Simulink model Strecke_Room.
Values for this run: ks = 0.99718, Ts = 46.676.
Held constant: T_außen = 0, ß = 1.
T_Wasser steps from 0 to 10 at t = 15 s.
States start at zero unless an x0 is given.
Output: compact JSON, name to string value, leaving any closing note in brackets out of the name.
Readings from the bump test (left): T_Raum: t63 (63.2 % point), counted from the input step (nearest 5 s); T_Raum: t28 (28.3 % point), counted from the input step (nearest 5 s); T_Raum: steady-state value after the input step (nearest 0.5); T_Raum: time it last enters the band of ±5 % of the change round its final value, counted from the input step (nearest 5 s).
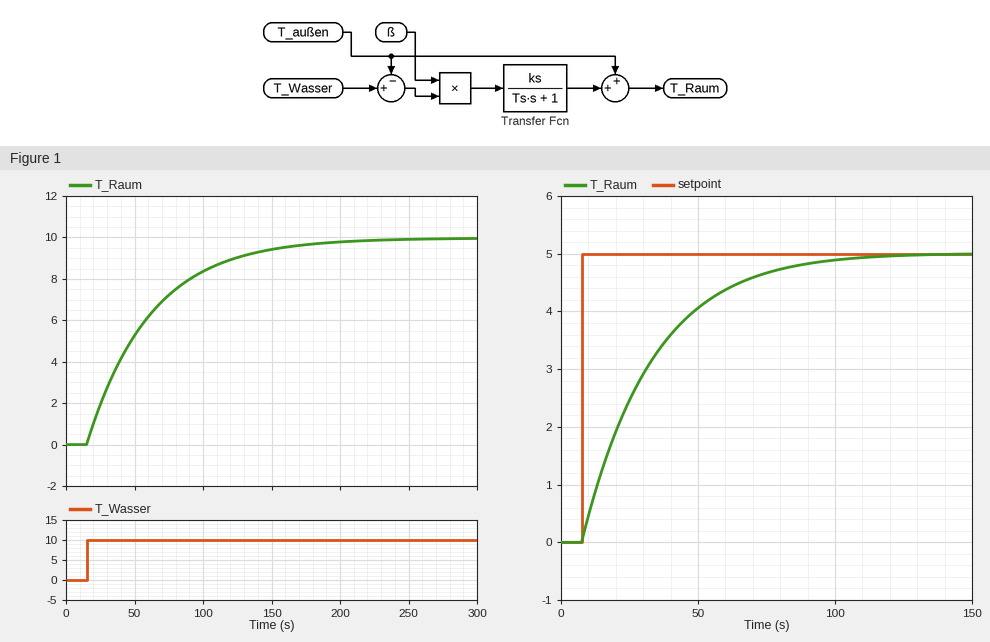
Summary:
{"T_Raum: t63 (63.2 % point), counted from the input step": "45 s", "T_Raum: t28 (28.3 % point), counted from the input step": "15 s", "T_Raum: steady-state value after the input step": "10.0", "T_Raum: time it last enters the band of ±5 % of the change round its final value, counted from the input step": "140 s"}
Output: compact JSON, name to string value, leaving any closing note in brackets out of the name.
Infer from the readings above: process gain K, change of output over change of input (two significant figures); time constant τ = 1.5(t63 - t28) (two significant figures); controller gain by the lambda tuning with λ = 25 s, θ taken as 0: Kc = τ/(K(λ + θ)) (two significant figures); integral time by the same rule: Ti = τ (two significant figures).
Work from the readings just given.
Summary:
{"process gain K, change of output over change of input": "1.0", "time constant τ = 1.5(t63 - t28)": "45 s", "controller gain by the lambda tuning with λ = 25 s, θ taken as 0: Kc = τ/(K(λ + θ))": "1.8", "integral time by the same rule: Ti = τ": "45 s"}
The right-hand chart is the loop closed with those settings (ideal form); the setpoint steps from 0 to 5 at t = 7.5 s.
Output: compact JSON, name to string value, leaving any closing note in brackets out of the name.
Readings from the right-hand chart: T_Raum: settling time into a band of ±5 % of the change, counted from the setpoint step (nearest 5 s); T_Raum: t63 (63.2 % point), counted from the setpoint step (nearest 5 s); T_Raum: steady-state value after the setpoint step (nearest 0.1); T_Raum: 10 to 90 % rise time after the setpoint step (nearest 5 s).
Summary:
{"T_Raum: settling time into a band of ±5 % of the change, counted from the setpoint step": "75 s", "T_Raum: t63 (63.2 % point), counted from the setpoint step": "25 s", "T_Raum: steady-state value after the setpoint step": "5.0", "T_Raum: 10 to 90 % rise time after the setpoint step": "55 s"}
